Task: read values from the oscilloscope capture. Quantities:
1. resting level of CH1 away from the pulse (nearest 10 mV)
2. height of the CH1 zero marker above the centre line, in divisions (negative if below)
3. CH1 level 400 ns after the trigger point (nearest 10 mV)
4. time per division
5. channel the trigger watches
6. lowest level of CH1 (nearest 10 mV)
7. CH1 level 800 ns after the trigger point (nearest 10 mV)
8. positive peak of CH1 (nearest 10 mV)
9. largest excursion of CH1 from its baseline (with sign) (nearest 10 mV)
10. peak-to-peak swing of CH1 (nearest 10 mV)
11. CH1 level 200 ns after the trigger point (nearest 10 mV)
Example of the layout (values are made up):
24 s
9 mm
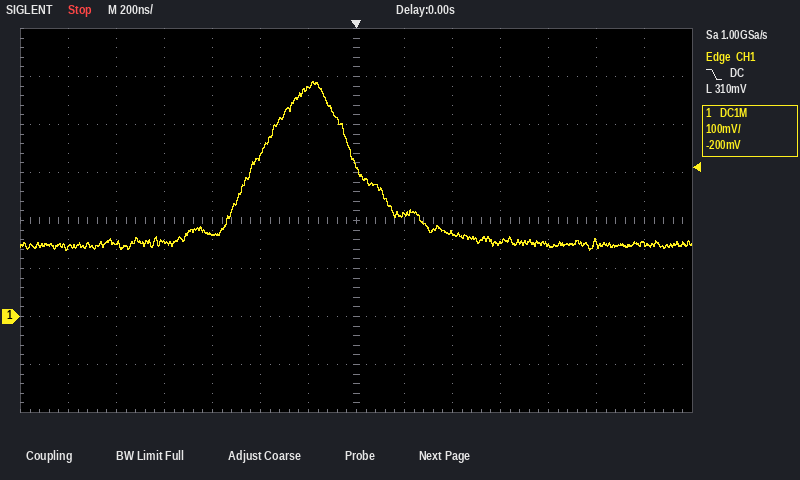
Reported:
150 mV
-2.0 div
170 mV
200 ns
CH1
140 mV
150 mV
490 mV
+340 mV
350 mV
210 mV
